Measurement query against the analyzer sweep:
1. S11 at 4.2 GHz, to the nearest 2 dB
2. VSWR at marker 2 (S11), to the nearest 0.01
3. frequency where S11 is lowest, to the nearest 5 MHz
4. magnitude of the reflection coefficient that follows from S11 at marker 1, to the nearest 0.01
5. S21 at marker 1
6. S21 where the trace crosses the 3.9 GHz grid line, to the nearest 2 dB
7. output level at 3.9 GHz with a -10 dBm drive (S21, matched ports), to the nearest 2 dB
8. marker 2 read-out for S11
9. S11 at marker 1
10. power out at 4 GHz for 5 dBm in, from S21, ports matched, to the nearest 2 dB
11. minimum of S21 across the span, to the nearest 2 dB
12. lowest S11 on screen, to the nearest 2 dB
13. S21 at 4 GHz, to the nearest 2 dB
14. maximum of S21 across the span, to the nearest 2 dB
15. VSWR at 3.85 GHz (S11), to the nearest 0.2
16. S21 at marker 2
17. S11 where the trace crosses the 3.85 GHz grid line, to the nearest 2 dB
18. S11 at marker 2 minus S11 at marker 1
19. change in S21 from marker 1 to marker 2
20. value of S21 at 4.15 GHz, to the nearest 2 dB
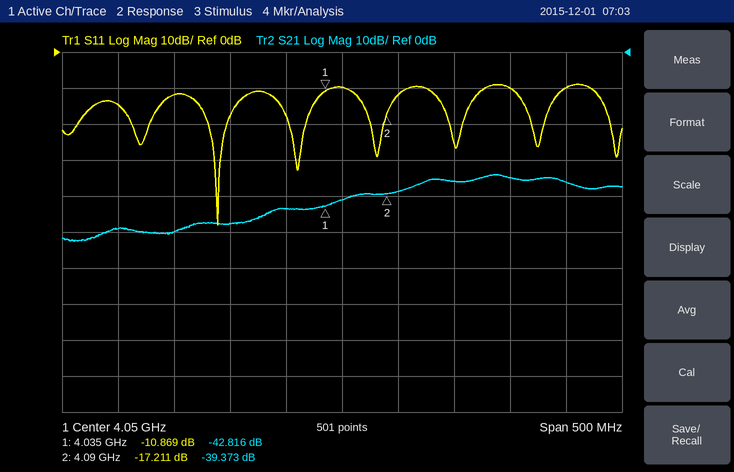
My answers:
-10 dB
1.32
3.940 GHz
0.29
-42.816 dB
-50 dB
-60 dBm
-17.211 dB
-10.869 dB
-38 dBm
-52 dB
-48 dB
-44 dB
-34 dB
1.4
-39.373 dB
-14 dB
-6.342 dB
3.443 dB
-36 dB
